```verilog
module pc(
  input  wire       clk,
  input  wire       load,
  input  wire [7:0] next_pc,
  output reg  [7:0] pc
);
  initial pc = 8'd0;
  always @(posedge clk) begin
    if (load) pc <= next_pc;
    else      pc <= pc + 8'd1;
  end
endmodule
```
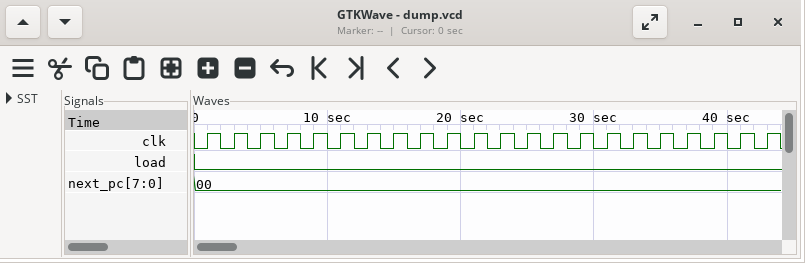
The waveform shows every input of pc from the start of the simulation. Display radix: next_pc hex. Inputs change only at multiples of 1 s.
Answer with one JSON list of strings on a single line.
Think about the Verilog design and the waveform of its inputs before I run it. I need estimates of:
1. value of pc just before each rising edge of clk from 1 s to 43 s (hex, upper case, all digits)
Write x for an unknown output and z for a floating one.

["00, 01, 02, 03, 04, 05, 06, 07, 08, 09, 0A, 0B, 0C, 0D, 0E, 0F, 10, 11, 12, 13, 14, 15"]
